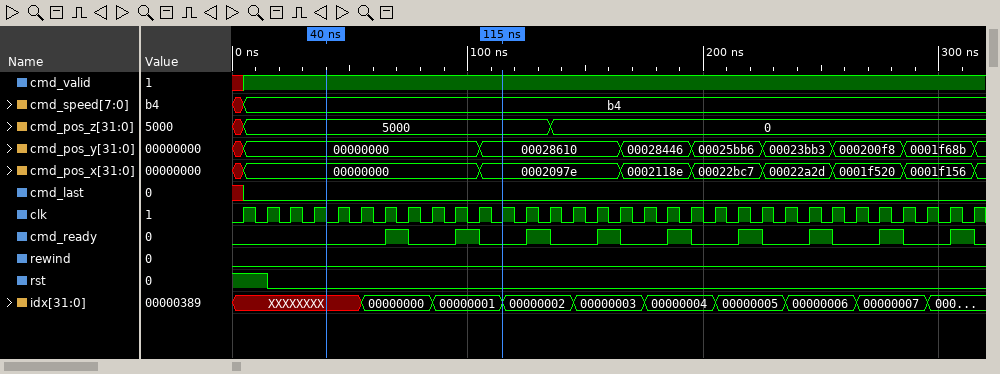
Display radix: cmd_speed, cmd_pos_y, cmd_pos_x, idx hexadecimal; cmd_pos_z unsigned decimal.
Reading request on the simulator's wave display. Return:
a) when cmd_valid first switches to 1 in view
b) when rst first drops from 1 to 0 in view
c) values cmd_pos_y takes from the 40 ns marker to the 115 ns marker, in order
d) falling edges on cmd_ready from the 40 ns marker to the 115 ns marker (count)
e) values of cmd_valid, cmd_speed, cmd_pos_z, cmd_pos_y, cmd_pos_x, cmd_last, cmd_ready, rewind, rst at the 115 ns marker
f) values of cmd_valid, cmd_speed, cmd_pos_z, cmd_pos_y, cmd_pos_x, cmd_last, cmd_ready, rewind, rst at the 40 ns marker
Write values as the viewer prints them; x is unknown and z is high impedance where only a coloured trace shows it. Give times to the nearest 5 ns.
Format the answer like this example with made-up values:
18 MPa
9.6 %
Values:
5 ns
15 ns
00000000, 00028610
2
cmd_valid=1, cmd_speed=b4, cmd_pos_z=5000, cmd_pos_y=00028610, cmd_pos_x=0002097e, cmd_last=0, cmd_ready=0, rewind=0, rst=0
cmd_valid=1, cmd_speed=b4, cmd_pos_z=5000, cmd_pos_y=00000000, cmd_pos_x=00000000, cmd_last=0, cmd_ready=0, rewind=0, rst=0
